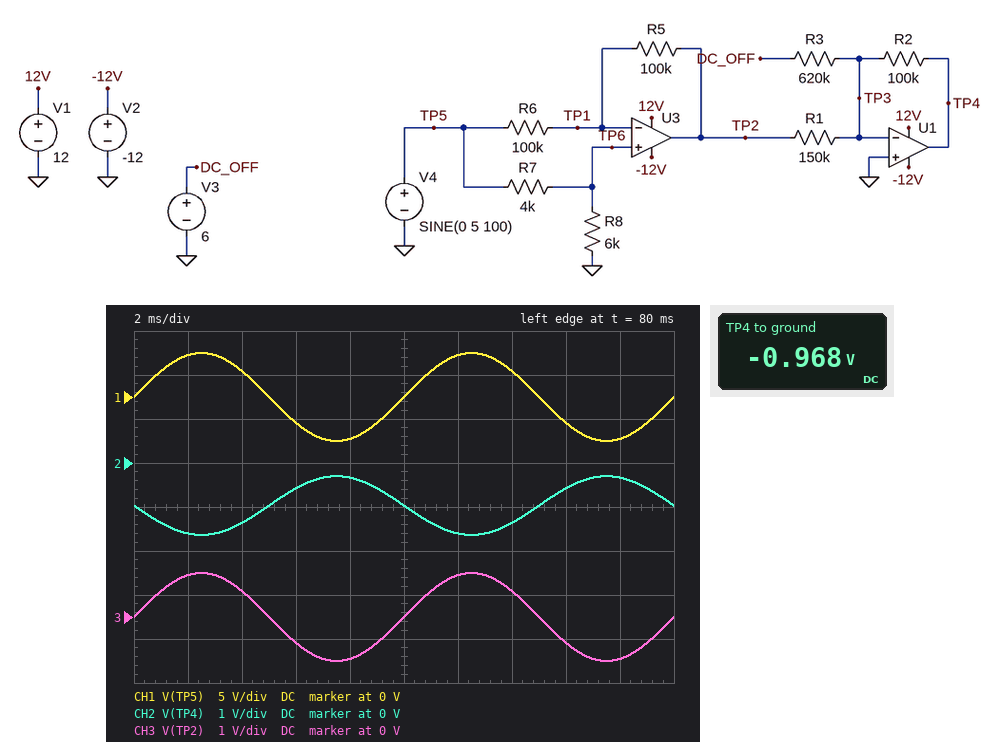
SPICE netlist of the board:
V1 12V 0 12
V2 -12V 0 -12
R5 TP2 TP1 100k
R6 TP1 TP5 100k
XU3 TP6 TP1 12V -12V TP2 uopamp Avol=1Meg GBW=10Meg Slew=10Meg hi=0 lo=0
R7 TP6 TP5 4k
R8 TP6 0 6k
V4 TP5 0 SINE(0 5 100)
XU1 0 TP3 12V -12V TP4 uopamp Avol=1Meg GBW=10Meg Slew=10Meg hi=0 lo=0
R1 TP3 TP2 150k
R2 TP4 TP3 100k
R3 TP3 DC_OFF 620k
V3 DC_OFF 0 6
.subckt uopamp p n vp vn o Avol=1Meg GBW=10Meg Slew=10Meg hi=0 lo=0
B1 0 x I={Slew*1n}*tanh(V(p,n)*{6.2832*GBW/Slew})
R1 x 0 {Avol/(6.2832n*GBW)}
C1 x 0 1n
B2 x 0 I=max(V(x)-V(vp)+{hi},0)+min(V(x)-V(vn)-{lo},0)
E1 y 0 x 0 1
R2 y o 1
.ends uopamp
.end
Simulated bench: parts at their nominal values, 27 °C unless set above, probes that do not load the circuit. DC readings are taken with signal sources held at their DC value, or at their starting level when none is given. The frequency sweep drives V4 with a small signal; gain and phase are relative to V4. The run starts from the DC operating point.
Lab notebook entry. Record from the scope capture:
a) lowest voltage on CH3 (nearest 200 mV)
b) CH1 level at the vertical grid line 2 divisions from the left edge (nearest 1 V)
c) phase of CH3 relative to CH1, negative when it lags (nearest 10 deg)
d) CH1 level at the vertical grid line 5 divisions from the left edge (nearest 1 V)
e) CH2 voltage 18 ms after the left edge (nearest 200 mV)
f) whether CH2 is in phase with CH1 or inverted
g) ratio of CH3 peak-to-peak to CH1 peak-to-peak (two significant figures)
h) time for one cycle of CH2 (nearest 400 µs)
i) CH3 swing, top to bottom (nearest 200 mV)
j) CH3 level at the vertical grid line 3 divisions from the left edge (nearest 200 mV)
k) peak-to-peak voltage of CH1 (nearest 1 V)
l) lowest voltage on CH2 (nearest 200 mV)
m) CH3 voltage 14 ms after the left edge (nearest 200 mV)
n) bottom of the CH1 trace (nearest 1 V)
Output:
-1.0 V
3 V
0 deg
0 V
-400 mV
inverted
0.20
10.0 ms
2.0 V
-600 mV
10 V
-1.6 V
600 mV
-5 V
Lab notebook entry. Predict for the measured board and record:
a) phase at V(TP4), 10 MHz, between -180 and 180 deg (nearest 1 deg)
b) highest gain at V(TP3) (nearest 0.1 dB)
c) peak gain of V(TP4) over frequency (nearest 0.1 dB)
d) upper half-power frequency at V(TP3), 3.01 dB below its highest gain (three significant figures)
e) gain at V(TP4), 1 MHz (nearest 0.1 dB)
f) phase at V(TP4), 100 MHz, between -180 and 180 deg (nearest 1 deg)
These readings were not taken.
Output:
55 deg
-29.2 dB
-17.5 dB
12.6 MHz
-17.8 dB
6 deg
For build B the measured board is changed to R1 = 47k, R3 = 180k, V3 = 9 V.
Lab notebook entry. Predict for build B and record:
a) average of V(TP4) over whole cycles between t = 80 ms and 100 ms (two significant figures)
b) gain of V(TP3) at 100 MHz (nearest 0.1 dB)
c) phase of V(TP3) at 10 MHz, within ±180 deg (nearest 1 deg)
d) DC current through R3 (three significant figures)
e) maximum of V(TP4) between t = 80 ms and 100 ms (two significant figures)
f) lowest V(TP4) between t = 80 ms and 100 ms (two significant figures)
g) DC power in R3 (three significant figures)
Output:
-5.0 V
-44.8 dB
-48 deg
50.0 µA
-2.9 V
-7.1 V
450 µW
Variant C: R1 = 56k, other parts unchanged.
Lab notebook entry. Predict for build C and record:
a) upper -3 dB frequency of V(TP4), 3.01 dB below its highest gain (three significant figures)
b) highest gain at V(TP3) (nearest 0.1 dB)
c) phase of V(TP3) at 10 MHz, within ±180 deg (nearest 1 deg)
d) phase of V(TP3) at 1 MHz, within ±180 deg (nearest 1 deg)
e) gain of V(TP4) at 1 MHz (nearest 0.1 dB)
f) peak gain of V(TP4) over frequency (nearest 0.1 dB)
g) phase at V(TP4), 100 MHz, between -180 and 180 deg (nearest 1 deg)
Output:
2.58 MHz
-22.8 dB
-45 deg
62 deg
-9.5 dB
-8.9 dB
5 deg
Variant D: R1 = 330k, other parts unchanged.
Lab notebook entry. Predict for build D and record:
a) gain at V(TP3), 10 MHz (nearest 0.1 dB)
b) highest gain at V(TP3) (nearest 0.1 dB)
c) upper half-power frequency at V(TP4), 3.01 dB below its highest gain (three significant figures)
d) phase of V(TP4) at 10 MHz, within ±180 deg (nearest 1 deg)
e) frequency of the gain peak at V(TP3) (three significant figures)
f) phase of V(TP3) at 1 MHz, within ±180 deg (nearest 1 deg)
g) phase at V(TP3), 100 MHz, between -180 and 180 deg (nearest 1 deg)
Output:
-36.3 dB
-35.1 dB
3.70 MHz
61 deg
5.84 MHz
70 deg
-83 deg
